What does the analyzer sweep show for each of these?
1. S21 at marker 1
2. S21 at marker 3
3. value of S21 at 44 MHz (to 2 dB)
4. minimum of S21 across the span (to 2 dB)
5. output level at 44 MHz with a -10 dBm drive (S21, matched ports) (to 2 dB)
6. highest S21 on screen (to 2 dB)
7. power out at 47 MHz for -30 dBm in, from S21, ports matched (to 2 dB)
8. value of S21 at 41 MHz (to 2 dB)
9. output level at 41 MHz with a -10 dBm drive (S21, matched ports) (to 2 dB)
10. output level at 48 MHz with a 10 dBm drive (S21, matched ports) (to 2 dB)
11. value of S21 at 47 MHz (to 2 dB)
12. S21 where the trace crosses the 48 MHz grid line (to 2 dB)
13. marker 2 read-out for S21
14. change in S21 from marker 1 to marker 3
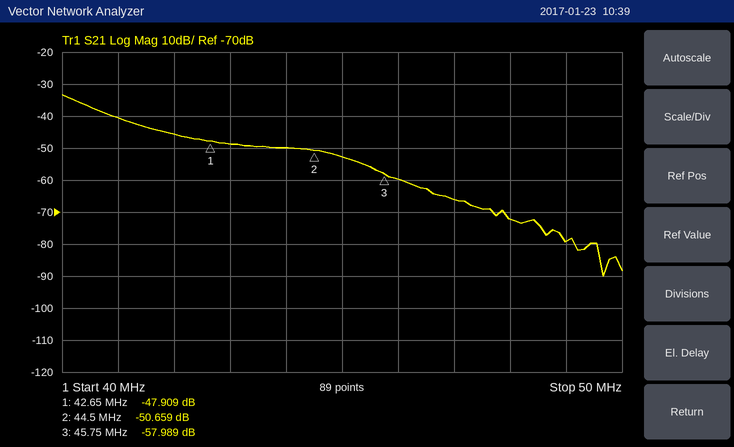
-47.909 dB
-57.989 dB
-50 dB
-90 dB
-60 dBm
-34 dB
-96 dBm
-40 dB
-50 dBm
-62 dBm
-66 dB
-72 dB
-50.659 dB
-10.080 dB
